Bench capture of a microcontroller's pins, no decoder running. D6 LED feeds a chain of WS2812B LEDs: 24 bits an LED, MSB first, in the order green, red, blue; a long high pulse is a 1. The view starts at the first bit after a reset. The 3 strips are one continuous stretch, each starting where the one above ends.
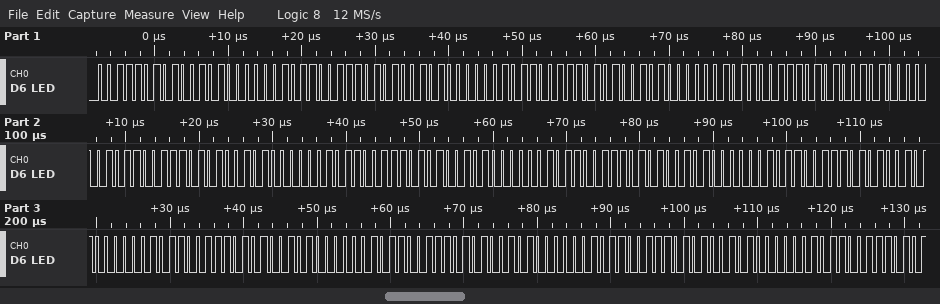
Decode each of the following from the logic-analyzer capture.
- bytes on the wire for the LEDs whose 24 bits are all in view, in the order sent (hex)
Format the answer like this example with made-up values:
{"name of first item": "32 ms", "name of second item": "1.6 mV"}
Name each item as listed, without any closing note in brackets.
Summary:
{"bytes on the wire for the LEDs whose 24 bits are all in view, in the order sent": "3A 94 0B 3A 94 0B 3A 94 0B 3A 94 0B 3A 94 0B 3A 94 0B 3A 94 0B 3A 94 0B 3A 94 0B 3A 94 0B 3A 94 0B"}
